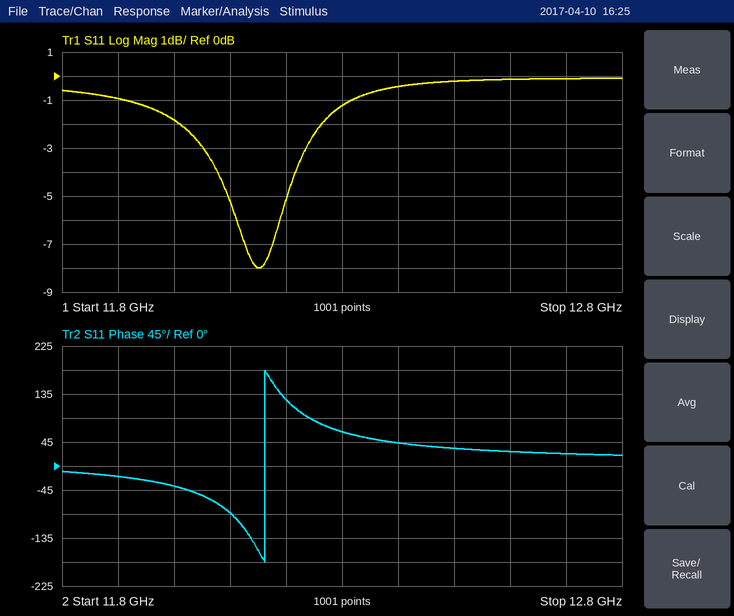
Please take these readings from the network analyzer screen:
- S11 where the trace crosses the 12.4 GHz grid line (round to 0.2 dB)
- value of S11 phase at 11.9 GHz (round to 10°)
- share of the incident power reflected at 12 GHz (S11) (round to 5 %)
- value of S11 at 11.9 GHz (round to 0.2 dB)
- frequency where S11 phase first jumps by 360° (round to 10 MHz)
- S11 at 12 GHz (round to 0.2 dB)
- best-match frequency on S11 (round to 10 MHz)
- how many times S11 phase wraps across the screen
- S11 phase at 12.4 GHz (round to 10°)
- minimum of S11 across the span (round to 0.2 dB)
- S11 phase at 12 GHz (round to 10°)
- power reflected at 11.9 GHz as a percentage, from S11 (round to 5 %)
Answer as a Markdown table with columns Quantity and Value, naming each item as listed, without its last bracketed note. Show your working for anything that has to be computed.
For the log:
| Quantity | Value |
|---|---|
| S11 where the trace crosses the 12.4 GHz grid line | -0.4 dB |
| value of S11 phase at 11.9 GHz | -20° |
| share of the incident power reflected at 12 GHz (S11) | 10^(-1.8/10) ≈ 66.1 %, so 65 % to the nearest 5 % |
| value of S11 at 11.9 GHz | -1.0 dB |
| frequency where S11 phase first jumps by 360° | 12.16 GHz |
| S11 at 12 GHz | -1.8 dB |
| best-match frequency on S11 | 12.15 GHz |
| how many times S11 phase wraps across the screen | 1 |
| S11 phase at 12.4 GHz | 40° |
| minimum of S11 across the span | -8.0 dB |
| S11 phase at 12 GHz | -40° |
| power reflected at 11.9 GHz as a percentage, from S11 | 10^(-1/10) ≈ 79.4 %, so 80 % to the nearest 5 % |
